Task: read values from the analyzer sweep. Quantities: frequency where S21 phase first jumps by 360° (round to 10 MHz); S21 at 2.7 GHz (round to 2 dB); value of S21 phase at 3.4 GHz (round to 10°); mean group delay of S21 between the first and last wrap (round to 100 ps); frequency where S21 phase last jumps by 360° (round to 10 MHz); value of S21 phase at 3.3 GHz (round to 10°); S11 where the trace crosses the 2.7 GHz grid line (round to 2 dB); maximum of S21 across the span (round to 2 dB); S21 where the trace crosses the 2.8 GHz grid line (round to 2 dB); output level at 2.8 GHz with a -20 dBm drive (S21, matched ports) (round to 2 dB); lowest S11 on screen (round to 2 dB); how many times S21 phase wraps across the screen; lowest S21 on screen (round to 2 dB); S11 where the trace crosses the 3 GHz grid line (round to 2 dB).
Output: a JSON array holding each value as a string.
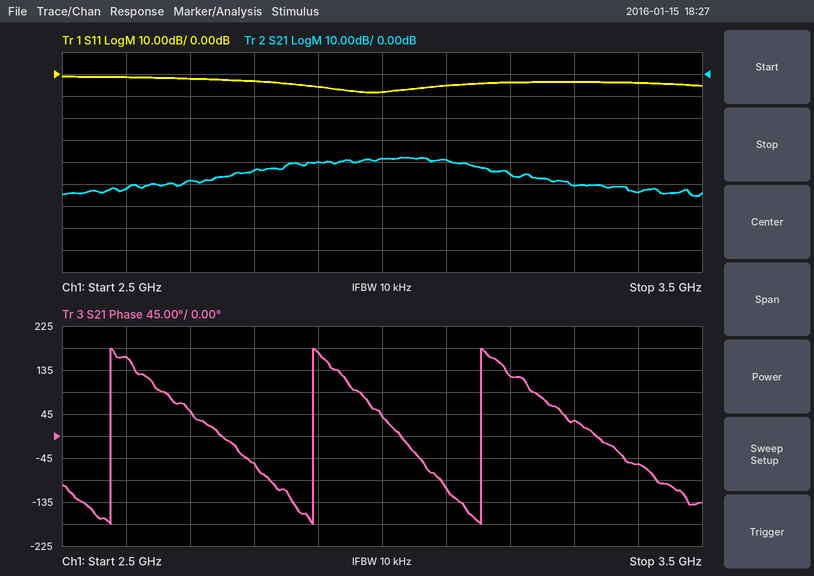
["2.58 GHz", "-48 dB", "-60°", "3.5 ns", "3.15 GHz", "30°", "-2 dB", "-38 dB", "-44 dB", "-64 dBm", "-8 dB", "3", "-56 dB", "-8 dB"]
